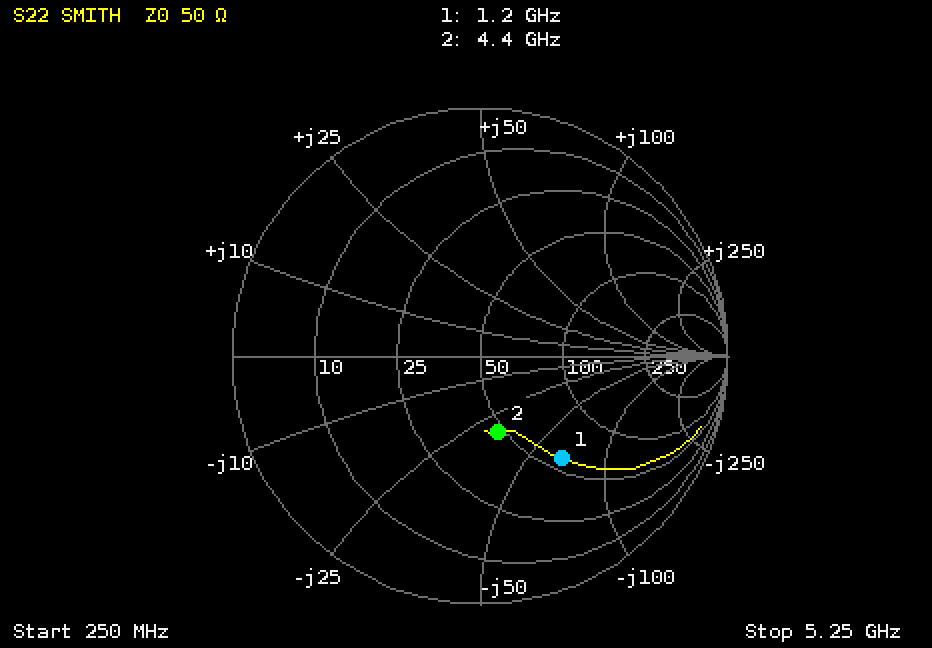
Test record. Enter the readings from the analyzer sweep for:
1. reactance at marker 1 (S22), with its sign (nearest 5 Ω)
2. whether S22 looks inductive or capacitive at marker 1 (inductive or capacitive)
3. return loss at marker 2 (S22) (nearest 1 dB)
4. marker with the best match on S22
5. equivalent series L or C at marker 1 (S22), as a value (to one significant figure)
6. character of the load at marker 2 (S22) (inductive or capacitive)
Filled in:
-65 Ω
capacitive
10 dB
marker 2
2 pF
capacitive
